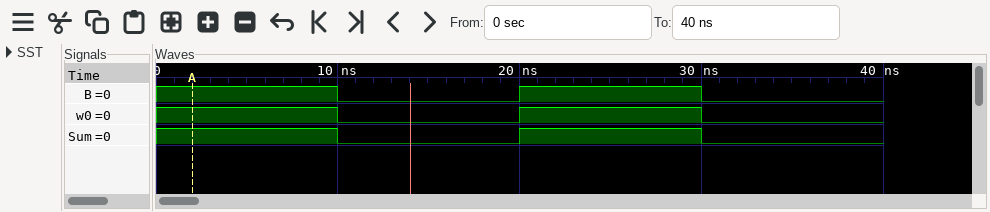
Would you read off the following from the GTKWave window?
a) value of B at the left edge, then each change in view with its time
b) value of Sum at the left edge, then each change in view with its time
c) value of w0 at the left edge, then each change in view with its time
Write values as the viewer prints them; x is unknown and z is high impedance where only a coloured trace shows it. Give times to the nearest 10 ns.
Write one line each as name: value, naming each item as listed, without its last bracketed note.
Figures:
value of B at the left edge, then each change in view with its time: 1, 0 at 10 ns, 1 at 20 ns, 0 at 30 ns
value of Sum at the left edge, then each change in view with its time: 1, 0 at 10 ns, 1 at 20 ns, 0 at 30 ns
value of w0 at the left edge, then each change in view with its time: 1, 0 at 10 ns, 1 at 20 ns, 0 at 30 ns
